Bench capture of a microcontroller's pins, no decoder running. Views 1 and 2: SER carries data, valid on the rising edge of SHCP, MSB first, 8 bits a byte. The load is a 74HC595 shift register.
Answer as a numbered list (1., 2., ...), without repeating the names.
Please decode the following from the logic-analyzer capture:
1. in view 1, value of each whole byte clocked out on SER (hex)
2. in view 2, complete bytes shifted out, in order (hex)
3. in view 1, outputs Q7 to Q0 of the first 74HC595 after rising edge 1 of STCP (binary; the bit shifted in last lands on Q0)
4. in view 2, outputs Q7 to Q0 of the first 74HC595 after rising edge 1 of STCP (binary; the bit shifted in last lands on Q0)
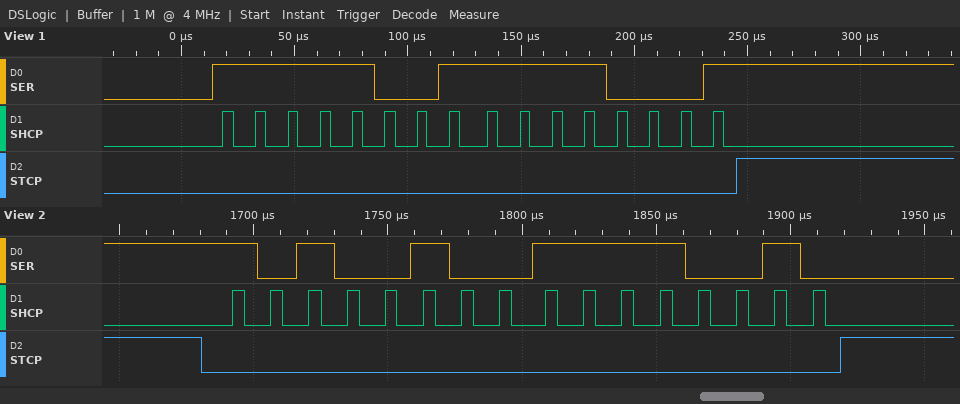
1. 0xF9 0xF1
2. A4 F2
3. 11110001
4. 11110010
